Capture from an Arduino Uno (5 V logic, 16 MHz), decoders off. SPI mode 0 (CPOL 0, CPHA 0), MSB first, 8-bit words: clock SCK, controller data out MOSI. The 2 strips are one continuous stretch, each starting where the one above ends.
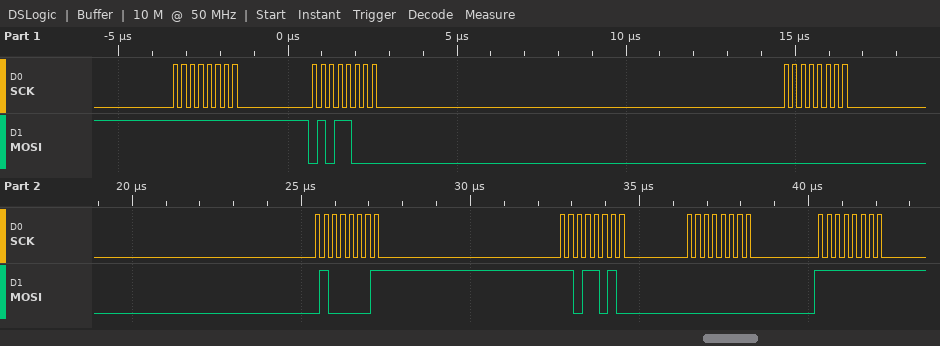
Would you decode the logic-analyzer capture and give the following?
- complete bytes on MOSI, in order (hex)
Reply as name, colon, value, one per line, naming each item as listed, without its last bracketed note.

complete bytes on MOSI, in order: FF 58 00 41 DA 00 FF
